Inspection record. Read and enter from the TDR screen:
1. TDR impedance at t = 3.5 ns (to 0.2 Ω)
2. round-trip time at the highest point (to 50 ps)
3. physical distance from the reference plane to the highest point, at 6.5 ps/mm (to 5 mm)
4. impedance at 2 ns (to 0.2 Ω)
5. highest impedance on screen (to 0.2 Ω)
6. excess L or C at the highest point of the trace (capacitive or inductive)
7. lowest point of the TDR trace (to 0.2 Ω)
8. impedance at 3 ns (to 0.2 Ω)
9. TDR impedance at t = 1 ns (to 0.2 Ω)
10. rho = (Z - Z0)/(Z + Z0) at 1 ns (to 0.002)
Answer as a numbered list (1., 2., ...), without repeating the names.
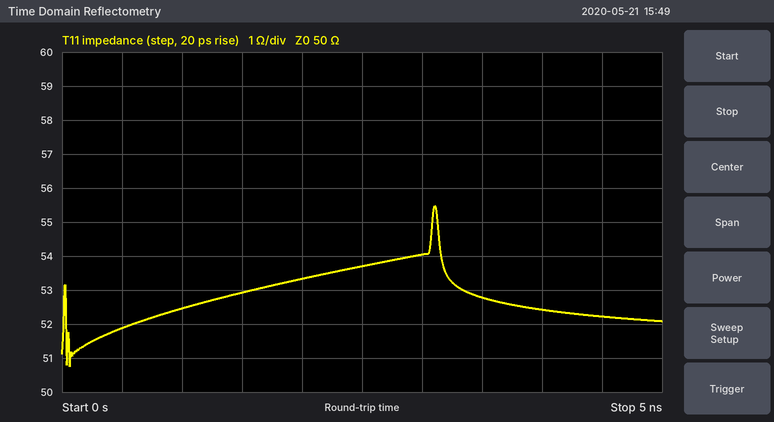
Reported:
1. 52.8 Ω
2. 3.10 ns
3. 240 mm
4. 53.4 Ω
5. 55.4 Ω
6. inductive
7. 50.8 Ω
8. 54.0 Ω
9. 52.4 Ω
10. +0.024
